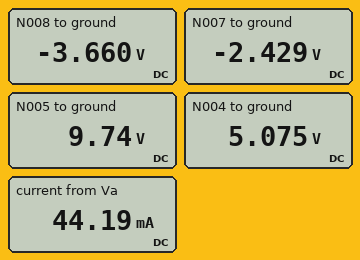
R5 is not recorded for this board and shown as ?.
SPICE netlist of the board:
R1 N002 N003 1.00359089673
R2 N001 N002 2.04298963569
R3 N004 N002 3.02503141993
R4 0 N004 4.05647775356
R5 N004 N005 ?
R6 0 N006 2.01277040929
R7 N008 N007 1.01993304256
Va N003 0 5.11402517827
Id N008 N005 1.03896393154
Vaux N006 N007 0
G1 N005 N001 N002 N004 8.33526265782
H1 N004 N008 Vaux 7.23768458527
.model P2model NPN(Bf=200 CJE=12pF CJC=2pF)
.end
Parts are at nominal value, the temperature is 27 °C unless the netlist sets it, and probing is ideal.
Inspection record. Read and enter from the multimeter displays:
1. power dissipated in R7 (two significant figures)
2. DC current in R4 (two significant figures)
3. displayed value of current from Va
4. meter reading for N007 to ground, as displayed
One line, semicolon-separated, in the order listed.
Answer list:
1.5 W; 1.3 A; 44.19 mA; -2.429 V
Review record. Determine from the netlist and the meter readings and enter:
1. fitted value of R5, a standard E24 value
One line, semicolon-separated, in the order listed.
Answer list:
4.3 Ω
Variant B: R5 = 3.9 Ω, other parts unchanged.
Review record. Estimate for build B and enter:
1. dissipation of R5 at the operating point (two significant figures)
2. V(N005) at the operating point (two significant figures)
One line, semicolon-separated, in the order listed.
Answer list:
4.6 W; 9.3 V
